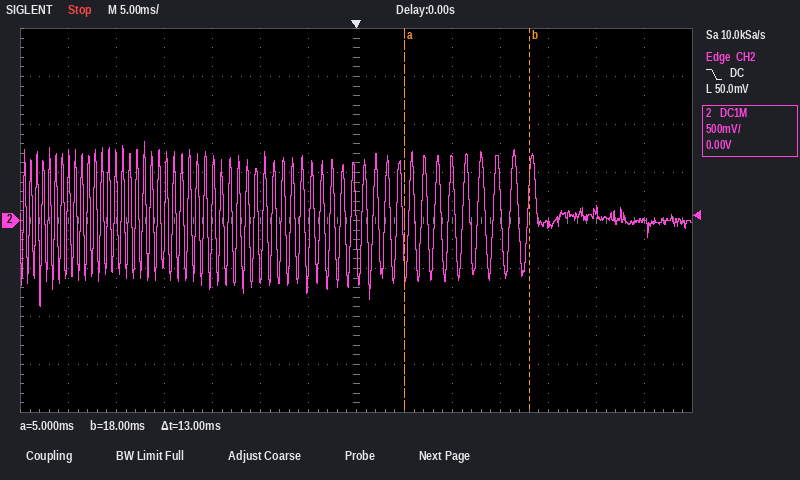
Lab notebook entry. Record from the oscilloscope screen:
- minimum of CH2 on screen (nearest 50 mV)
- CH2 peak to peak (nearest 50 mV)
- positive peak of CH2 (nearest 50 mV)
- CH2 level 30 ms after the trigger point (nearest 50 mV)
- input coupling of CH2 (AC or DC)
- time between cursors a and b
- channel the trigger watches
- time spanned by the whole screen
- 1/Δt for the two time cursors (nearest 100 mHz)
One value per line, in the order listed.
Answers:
-900 mV
1.70 V
800 mV
0 mV
DC
13 ms
CH2
70 ms
76.9 Hz
